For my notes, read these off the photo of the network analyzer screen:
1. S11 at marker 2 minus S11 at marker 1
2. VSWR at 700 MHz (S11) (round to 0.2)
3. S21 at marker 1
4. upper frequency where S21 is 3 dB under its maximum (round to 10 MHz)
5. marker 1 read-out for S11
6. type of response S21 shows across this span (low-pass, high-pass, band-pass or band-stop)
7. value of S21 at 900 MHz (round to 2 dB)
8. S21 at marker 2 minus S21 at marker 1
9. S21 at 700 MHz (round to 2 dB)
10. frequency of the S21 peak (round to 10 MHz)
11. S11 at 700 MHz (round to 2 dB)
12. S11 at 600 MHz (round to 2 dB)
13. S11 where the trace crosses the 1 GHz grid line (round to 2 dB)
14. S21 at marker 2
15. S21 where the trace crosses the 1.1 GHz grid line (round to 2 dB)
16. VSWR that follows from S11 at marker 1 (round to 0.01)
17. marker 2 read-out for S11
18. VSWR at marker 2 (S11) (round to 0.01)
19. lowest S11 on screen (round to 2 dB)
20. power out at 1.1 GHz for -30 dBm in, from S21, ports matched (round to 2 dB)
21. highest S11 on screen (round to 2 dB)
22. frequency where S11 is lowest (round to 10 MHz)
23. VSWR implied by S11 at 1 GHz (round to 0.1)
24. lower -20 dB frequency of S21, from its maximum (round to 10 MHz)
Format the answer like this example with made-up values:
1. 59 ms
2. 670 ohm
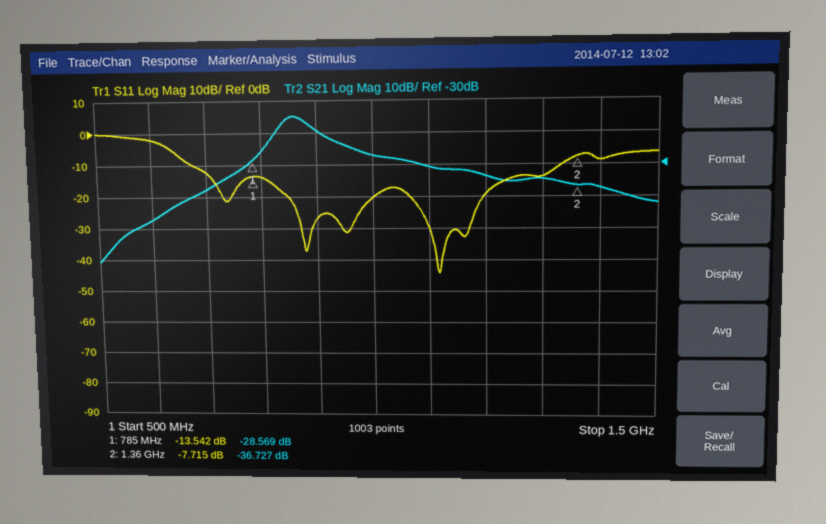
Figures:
1. 5.827 dB
2. 1.6
3. -28.569 dB
4. 890 MHz
5. -13.542 dB
6. band-pass
7. -20 dB
8. -8.158 dB
9. -38 dB
10. 860 MHz
11. -12 dB
12. -2 dB
13. -20 dB
14. -36.727 dB
15. -30 dB
16. 1.53
17. -7.715 dB
18. 2.40
19. -44 dB
20. -60 dBm
21. 0 dB
22. 1.12 GHz
23. 1.2
24. 730 MHz
